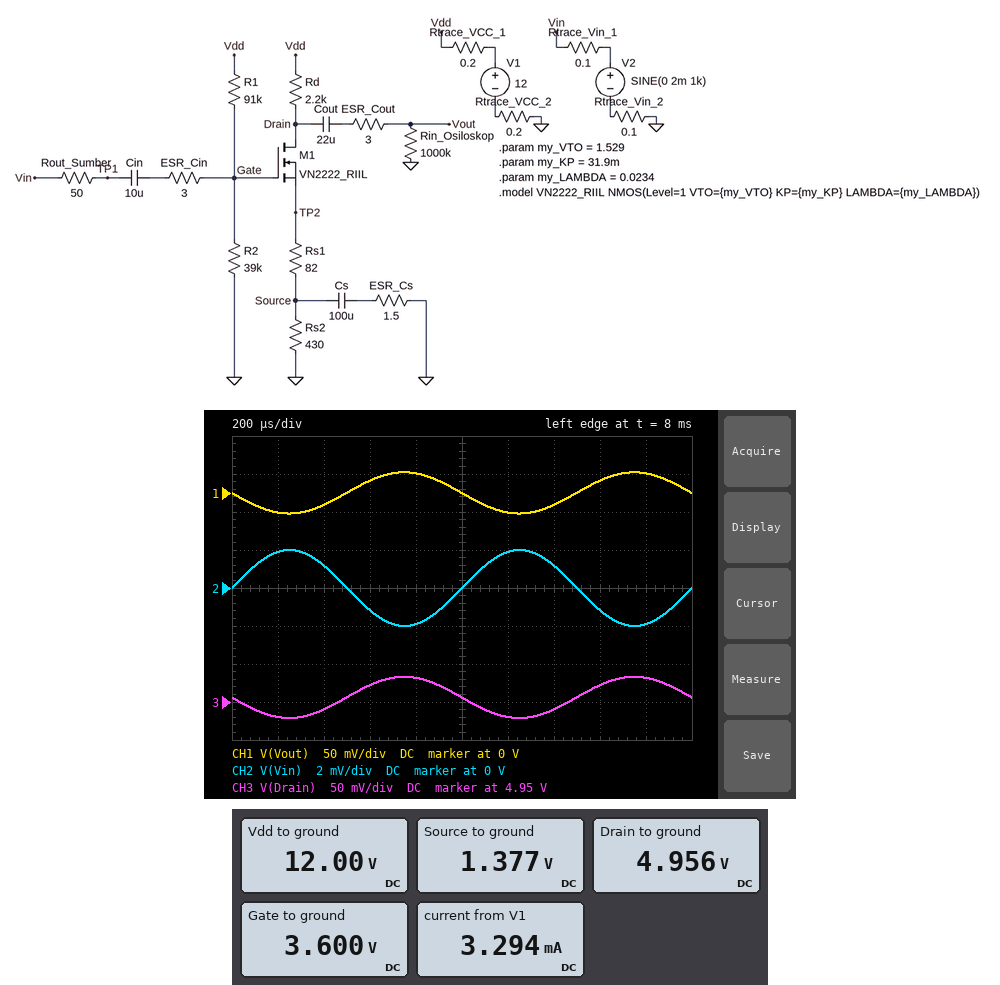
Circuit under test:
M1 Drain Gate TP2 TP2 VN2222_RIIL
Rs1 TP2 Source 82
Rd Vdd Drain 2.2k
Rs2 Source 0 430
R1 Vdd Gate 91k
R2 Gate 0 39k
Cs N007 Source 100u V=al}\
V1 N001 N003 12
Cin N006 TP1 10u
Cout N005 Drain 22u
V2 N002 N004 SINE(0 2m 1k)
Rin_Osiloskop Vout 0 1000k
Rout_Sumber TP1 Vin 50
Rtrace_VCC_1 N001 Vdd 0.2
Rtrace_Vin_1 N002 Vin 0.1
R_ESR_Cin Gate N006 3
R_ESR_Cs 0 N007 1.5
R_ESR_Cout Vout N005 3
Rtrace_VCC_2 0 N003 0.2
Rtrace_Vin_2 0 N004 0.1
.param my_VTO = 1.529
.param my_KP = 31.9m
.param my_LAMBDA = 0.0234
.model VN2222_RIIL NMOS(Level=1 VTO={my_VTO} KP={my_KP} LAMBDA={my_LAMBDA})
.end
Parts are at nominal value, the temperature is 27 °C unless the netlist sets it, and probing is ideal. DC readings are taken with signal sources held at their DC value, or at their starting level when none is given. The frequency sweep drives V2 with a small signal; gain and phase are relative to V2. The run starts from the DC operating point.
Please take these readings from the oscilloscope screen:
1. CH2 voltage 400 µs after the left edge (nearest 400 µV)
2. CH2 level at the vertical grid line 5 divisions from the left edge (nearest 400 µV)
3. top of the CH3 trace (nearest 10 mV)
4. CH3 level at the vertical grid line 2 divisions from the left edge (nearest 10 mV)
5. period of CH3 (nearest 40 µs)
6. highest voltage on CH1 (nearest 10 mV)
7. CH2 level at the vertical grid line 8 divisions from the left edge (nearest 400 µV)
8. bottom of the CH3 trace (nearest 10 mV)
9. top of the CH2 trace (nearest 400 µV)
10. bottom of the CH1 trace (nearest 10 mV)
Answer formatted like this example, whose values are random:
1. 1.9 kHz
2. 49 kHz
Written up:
1. 1.2 mV
2. 0 V
3. 4.98 V
4. 4.94 V
5. 1.00 ms
6. 30 mV
7. -1.2 mV
8. 4.93 V
9. 2.0 mV
10. -30 mV
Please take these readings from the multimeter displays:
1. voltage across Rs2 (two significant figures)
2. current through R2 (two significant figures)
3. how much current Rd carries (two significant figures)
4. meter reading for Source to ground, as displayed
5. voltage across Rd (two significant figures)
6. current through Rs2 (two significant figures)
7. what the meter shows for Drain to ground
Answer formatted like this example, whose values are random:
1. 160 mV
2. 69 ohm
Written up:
1. 1.4 V
2. 92 µA
3. 3.2 mA
4. 1.377 V
5. 7.0 V
6. 3.2 mA
7. 4.956 V
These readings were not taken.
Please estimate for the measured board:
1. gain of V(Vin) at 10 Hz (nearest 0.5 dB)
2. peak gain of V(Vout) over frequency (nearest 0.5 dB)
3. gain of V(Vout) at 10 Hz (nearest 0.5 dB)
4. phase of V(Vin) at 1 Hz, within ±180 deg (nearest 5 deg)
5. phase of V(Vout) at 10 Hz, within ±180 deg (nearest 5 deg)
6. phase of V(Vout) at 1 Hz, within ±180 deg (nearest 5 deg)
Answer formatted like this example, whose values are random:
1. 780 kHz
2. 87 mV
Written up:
1. 0 dB
2. 22.5 dB
3. 18.5 dB
4. 0 deg
5. -145 deg
6. -140 deg
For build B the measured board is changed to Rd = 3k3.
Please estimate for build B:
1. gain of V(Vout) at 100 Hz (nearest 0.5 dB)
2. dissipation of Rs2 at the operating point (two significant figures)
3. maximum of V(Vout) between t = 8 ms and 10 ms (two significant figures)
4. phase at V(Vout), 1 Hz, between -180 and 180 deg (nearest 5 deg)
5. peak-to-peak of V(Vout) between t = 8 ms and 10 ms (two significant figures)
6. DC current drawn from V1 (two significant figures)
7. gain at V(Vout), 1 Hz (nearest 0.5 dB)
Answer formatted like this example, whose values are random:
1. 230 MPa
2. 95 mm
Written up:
1. 0.5 dB
2. 4.1 mW
3. 2.1 mV
4. -145 deg
5. 4.2 mV
6. 3.2 mA
7. -3.0 dB
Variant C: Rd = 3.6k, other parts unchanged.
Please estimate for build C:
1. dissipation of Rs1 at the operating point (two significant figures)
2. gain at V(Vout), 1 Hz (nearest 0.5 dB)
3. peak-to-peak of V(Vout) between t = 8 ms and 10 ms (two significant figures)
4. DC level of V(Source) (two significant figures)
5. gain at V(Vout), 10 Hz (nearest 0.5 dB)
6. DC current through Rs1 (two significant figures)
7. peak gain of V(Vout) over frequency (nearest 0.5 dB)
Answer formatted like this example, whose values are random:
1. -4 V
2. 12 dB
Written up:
1. 680 µW
2. -10.5 dB
3. 1.6 mV
4. 1.2 V
5. -8.5 dB
6. 2.9 mA
7. -8.0 dB
